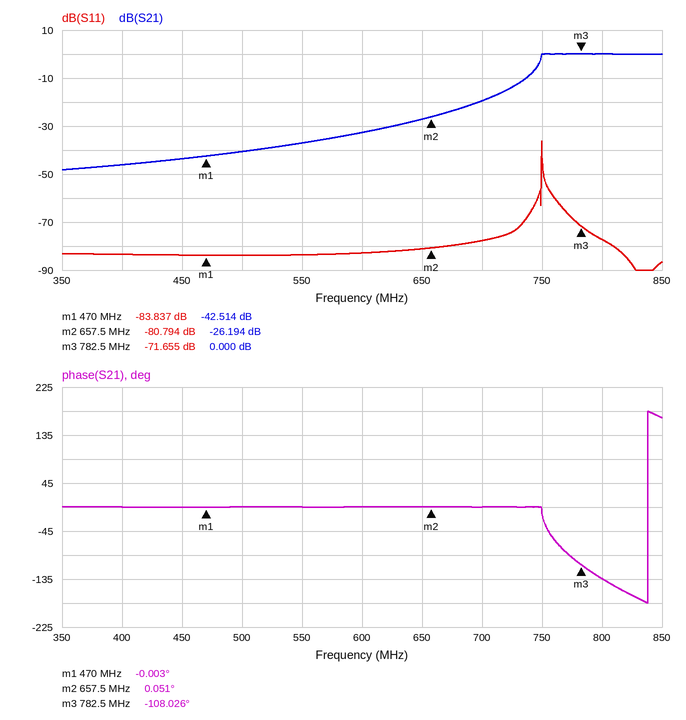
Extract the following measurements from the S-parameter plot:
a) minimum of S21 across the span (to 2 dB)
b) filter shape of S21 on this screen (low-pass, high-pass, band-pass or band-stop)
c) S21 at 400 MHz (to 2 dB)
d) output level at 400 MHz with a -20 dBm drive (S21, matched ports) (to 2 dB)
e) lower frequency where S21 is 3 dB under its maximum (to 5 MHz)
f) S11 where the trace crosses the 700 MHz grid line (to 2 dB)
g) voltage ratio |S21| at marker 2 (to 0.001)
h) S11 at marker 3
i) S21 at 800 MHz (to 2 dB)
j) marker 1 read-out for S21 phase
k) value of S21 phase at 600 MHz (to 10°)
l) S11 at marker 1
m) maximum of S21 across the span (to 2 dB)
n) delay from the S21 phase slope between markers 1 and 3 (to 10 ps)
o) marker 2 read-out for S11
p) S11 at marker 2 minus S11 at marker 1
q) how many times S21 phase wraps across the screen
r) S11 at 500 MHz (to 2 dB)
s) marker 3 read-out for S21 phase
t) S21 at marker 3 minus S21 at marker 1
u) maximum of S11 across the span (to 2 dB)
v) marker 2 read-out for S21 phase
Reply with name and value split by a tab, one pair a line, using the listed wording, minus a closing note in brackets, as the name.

minimum of S21 across the span	-48 dB
filter shape of S21 on this screen	high-pass
S21 at 400 MHz	-46 dB
output level at 400 MHz with a -20 dBm drive (S21, matched ports)	-66 dBm
lower frequency where S21 is 3 dB under its maximum	750 MHz
S11 where the trace crosses the 700 MHz grid line	-78 dB
voltage ratio |S21| at marker 2	0.049
S11 at marker 3	-71.655 dB
S21 at 800 MHz	0 dB
marker 1 read-out for S21 phase	-0.003°
value of S21 phase at 600 MHz	0°
S11 at marker 1	-83.837 dB
maximum of S21 across the span	0 dB
delay from the S21 phase slope between markers 1 and 3	960 ps
marker 2 read-out for S11	-80.794 dB
S11 at marker 2 minus S11 at marker 1	3.043 dB
how many times S21 phase wraps across the screen	1
S11 at 500 MHz	-84 dB
marker 3 read-out for S21 phase	-108.026°
S21 at marker 3 minus S21 at marker 1	42.514 dB
maximum of S11 across the span	-36 dB
marker 2 read-out for S21 phase	0.051°
